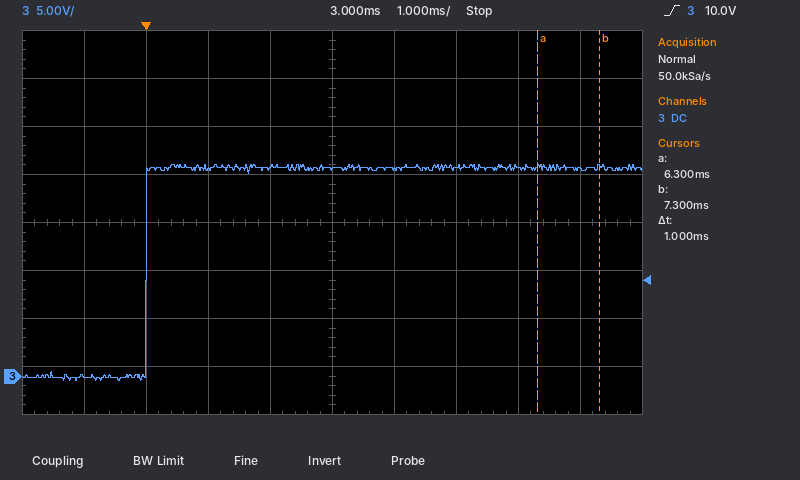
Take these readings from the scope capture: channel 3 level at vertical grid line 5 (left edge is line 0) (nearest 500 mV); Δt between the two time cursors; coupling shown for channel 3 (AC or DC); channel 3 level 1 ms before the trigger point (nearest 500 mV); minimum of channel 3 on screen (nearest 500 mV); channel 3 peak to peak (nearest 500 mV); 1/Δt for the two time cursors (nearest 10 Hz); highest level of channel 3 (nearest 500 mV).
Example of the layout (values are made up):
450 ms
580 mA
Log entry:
21.5 V
1 ms
DC
0.0 V
-500 mV
22.5 V
1.00 kHz
22.0 V
